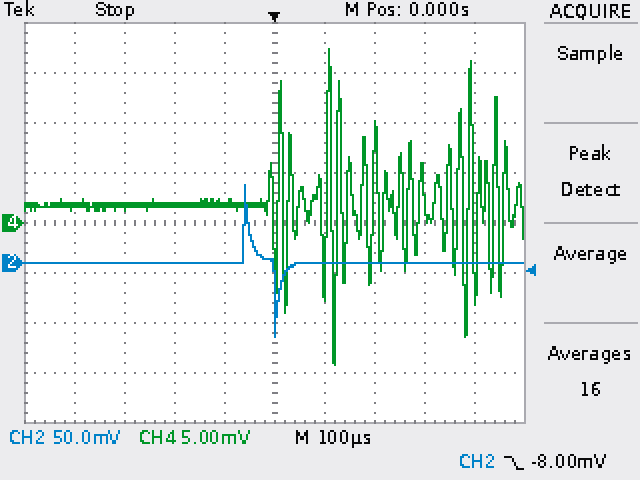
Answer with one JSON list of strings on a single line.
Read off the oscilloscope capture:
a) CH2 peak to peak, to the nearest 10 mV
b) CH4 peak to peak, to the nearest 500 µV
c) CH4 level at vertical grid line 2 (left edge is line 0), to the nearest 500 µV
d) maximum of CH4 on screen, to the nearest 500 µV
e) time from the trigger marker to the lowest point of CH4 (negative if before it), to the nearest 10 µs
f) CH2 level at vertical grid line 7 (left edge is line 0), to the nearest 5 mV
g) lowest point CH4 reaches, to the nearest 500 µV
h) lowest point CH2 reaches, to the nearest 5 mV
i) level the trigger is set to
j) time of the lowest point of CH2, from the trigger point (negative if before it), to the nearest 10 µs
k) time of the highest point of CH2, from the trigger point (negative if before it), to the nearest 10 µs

["150 mV", "31.5 mV", "1.5 mV", "17.5 mV", "+120 µs", "0 mV", "-14.0 mV", "-75 mV", "-8.00 mV", "0 µs", "-60 µs"]
